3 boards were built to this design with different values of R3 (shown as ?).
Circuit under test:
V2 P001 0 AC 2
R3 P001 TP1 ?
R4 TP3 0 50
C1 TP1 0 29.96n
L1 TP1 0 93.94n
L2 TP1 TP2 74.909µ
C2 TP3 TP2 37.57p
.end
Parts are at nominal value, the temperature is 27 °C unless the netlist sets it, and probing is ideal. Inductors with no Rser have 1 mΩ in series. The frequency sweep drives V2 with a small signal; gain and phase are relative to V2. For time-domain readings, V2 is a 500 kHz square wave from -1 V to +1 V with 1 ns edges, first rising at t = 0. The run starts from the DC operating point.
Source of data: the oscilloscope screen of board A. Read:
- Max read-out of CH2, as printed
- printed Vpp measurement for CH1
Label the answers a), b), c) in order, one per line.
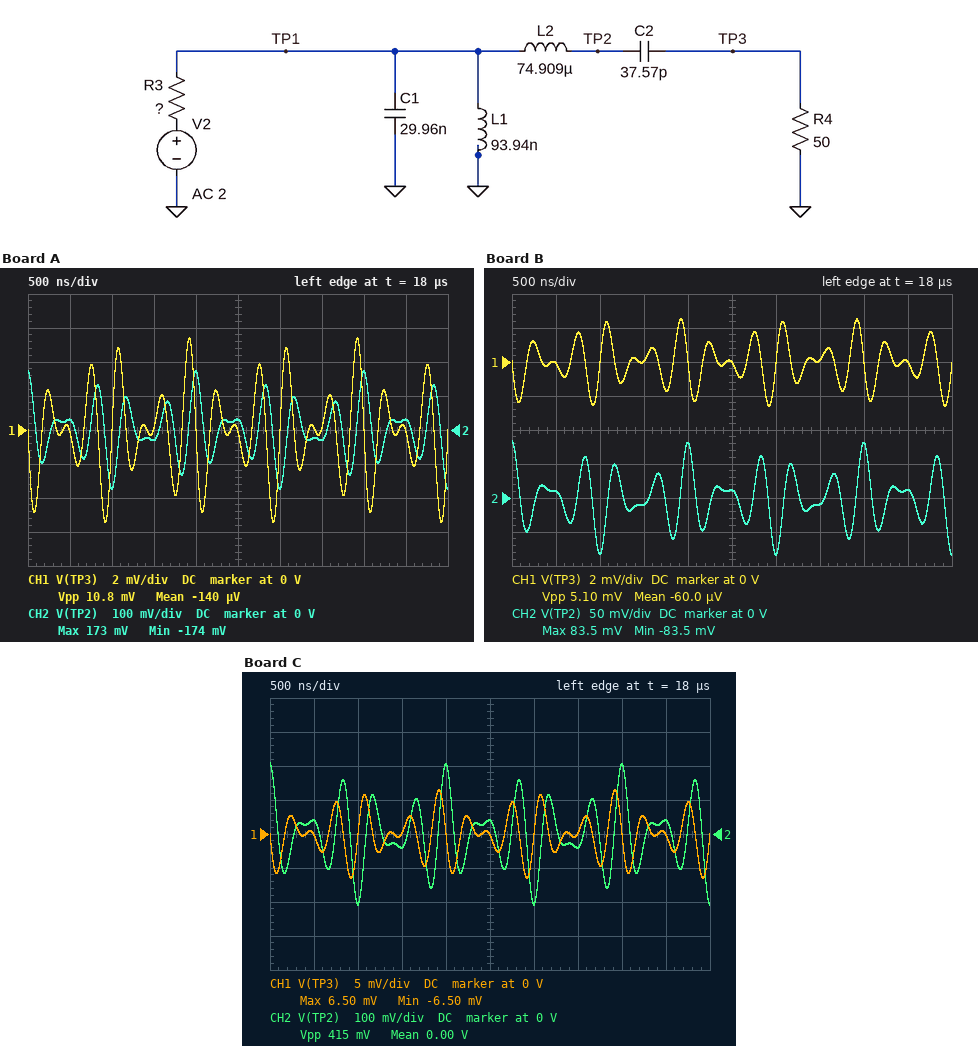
a) 173 mV
b) 10.8 mV
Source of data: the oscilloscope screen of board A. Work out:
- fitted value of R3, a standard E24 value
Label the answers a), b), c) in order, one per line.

a) 47 Ω
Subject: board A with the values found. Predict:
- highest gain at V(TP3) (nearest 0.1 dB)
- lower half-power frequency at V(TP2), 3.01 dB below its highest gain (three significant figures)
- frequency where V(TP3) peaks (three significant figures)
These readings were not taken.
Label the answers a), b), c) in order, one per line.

a) -5.8 dB
b) 2.92 MHz
c) 3.00 MHz
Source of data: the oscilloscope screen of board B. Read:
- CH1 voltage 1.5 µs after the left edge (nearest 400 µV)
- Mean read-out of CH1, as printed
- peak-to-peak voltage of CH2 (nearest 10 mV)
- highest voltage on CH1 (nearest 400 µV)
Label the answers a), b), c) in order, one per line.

a) 0 V
b) -60.0 µV
c) 170 mV
d) 2.4 mV
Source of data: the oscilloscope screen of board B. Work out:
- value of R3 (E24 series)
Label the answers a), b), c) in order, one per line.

a) 100 Ω
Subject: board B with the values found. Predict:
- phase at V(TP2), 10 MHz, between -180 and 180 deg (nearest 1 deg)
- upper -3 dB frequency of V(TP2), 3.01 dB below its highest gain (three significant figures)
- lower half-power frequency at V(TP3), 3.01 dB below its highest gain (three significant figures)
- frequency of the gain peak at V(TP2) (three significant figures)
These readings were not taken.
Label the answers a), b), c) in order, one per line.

a) 98 deg
b) 3.07 MHz
c) 2.93 MHz
d) 2.97 MHz
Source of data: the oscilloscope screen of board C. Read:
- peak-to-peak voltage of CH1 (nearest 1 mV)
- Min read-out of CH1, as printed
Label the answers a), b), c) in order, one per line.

a) 13 mV
b) -6.50 mV
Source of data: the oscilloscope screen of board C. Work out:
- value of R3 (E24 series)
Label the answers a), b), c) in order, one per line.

a) 39 Ω
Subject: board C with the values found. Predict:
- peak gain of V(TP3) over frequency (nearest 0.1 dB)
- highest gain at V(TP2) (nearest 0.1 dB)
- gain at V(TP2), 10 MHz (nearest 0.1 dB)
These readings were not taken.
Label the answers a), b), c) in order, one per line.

a) -5.1 dB
b) 24.0 dB
c) -56.5 dB
